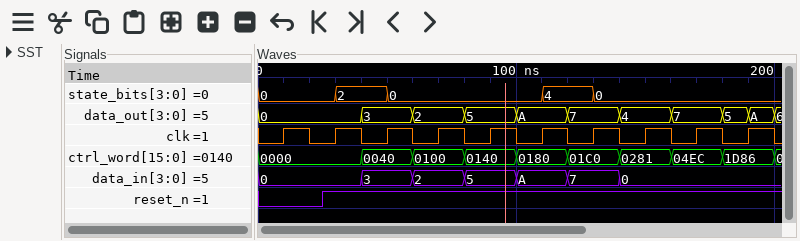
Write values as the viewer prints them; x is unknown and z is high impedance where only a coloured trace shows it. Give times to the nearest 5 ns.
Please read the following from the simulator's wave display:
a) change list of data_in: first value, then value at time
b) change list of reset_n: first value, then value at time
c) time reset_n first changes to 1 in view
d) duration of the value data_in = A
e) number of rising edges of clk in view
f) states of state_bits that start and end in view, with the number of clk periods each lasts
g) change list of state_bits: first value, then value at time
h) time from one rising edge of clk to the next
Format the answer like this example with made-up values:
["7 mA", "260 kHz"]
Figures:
["0, 3 at 40 ns, 2 at 60 ns, 5 at 80 ns, A at 100 ns, 7 at 120 ns, 0 at 140 ns", "0, 1 at 25 ns", "25 ns", "20 ns", "10", "2: 1, 0: 3, 4: 1", "0, 2 at 30 ns, 0 at 50 ns, 4 at 110 ns, 0 at 130 ns", "20 ns"]
